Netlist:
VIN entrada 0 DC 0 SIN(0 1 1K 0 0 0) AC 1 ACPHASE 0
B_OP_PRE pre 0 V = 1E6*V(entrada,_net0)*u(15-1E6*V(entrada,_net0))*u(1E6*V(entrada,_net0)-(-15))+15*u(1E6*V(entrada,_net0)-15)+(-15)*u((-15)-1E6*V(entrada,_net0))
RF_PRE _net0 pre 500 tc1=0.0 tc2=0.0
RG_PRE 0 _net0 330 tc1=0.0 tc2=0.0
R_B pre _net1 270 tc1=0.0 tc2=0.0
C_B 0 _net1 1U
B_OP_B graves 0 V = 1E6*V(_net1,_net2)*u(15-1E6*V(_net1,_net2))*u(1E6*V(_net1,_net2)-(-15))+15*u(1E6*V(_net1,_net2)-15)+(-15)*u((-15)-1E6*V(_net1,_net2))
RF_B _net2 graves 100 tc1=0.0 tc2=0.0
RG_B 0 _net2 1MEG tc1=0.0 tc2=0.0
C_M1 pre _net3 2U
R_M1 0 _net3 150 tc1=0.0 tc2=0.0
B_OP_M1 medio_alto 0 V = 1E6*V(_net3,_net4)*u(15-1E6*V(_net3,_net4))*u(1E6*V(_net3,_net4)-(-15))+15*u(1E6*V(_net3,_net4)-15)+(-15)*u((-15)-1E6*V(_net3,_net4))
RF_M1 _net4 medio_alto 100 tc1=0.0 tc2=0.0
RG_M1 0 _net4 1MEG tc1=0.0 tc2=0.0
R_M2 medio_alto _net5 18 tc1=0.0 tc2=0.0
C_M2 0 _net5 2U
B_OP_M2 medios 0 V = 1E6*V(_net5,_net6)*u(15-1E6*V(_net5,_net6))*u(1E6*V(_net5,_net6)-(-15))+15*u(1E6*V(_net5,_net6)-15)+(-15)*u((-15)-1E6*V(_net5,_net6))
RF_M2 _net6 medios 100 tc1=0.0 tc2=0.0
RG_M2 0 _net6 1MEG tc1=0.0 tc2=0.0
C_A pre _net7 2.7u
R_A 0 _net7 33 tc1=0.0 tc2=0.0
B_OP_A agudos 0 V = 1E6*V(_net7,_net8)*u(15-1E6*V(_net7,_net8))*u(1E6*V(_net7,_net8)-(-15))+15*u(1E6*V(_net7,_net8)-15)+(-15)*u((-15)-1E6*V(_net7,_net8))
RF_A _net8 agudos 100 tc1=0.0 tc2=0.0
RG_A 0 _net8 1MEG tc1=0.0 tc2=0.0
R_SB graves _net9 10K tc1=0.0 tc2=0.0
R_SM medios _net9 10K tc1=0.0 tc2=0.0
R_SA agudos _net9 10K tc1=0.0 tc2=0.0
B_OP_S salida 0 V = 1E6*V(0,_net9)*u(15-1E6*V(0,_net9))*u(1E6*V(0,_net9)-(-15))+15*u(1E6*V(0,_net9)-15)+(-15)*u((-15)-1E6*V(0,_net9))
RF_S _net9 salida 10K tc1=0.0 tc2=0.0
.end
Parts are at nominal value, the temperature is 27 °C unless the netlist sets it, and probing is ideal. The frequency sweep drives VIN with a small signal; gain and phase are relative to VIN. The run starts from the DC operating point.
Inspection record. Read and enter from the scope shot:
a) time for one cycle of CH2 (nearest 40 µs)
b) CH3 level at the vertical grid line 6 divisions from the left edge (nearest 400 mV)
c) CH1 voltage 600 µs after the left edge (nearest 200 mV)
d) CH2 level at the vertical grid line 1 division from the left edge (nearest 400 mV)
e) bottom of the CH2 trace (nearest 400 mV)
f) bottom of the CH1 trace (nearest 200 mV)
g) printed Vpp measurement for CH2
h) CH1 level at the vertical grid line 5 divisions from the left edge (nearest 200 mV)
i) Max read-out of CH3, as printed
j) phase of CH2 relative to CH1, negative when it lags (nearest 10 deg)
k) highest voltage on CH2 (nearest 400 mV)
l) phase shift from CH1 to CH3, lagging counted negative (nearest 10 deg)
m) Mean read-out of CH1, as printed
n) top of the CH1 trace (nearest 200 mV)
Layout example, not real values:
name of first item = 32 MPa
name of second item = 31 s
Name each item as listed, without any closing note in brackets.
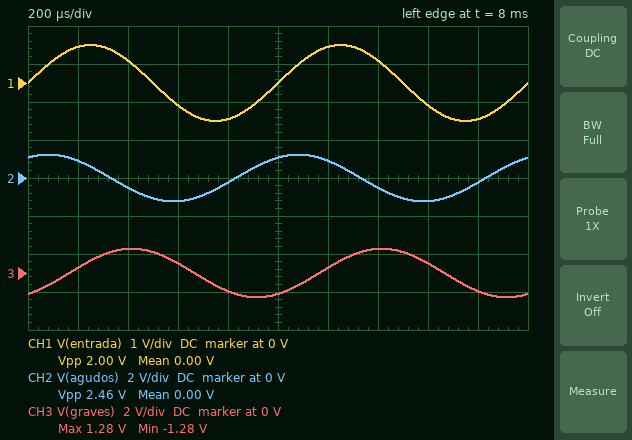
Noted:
time for one cycle of CH2 = 1.00 ms
CH3 level at the vertical grid line 6 divisions from the left edge = 400 mV
CH1 voltage 600 µs after the left edge = -600 mV
CH2 level at the vertical grid line 1 division from the left edge = 800 mV
bottom of the CH2 trace = -1.2 V
bottom of the CH1 trace = -1.0 V
printed Vpp measurement for CH2 = 2.46 V
CH1 level at the vertical grid line 5 divisions from the left edge = 0 V
Max read-out of CH3, as printed = 1.28 V
phase of CH2 relative to CH1, negative when it lags = 60 deg
highest voltage on CH2 = 1.2 V
phase shift from CH1 to CH3, lagging counted negative = -60 deg
Mean read-out of CH1, as printed = 0.00 V
top of the CH1 trace = 1.0 V
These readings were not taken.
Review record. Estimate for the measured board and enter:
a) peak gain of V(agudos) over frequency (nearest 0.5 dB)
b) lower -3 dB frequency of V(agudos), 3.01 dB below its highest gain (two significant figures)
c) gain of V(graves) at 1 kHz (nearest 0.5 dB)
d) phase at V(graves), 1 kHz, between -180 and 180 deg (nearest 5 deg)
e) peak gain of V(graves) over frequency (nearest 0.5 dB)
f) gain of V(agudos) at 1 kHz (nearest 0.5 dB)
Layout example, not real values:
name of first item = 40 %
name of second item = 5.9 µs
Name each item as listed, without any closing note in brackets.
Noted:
peak gain of V(agudos) over frequency = 8.0 dB
lower -3 dB frequency of V(agudos), 3.01 dB below its highest gain = 1.8 kHz
gain of V(graves) at 1 kHz = 2.0 dB
phase at V(graves), 1 kHz, between -180 and 180 deg = -60 deg
peak gain of V(graves) over frequency = 8.0 dB
gain of V(agudos) at 1 kHz = 2.0 dB
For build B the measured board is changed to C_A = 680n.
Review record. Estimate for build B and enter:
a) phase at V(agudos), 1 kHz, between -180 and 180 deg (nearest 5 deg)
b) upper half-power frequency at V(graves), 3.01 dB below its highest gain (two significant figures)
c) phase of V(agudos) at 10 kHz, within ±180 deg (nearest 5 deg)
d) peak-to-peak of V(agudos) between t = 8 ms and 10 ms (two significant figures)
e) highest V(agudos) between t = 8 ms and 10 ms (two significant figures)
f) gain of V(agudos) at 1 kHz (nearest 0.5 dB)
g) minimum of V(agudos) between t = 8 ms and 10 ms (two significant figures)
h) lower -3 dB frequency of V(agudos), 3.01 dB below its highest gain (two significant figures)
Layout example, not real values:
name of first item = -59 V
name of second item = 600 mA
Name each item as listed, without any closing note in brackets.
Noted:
phase at V(agudos), 1 kHz, between -180 and 180 deg = 80 deg
upper half-power frequency at V(graves), 3.01 dB below its highest gain = 590 Hz
phase of V(agudos) at 10 kHz, within ±180 deg = 35 deg
peak-to-peak of V(agudos) between t = 8 ms and 10 ms = 700 mV
highest V(agudos) between t = 8 ms and 10 ms = 350 mV
gain of V(agudos) at 1 kHz = -9.0 dB
minimum of V(agudos) between t = 8 ms and 10 ms = -350 mV
lower -3 dB frequency of V(agudos), 3.01 dB below its highest gain = 7.1 kHz
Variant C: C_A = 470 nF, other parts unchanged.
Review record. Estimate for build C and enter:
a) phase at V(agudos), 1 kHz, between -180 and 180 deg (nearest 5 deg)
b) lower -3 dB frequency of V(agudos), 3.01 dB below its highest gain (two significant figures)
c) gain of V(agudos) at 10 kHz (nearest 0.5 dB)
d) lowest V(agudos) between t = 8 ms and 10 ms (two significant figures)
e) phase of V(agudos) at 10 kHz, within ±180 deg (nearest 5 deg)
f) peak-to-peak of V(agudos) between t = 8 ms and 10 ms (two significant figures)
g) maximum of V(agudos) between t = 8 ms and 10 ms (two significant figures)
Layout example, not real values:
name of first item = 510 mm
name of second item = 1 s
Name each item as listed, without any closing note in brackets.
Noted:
phase at V(agudos), 1 kHz, between -180 and 180 deg = 85 deg
lower -3 dB frequency of V(agudos), 3.01 dB below its highest gain = 10 kHz
gain of V(agudos) at 10 kHz = 5.0 dB
lowest V(agudos) between t = 8 ms and 10 ms = -240 mV
phase of V(agudos) at 10 kHz, within ±180 deg = 45 deg
peak-to-peak of V(agudos) between t = 8 ms and 10 ms = 490 mV
maximum of V(agudos) between t = 8 ms and 10 ms = 240 mV
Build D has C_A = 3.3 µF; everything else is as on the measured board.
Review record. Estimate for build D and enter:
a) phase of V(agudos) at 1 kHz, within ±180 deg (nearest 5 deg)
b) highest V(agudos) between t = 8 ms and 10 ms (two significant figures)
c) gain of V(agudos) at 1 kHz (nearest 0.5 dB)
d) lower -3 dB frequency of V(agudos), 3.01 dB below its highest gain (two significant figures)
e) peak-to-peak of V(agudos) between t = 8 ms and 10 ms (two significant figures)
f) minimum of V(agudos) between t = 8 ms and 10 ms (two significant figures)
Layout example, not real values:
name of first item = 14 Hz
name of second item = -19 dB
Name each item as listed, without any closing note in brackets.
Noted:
phase of V(agudos) at 1 kHz, within ±180 deg = 55 deg
highest V(agudos) between t = 8 ms and 10 ms = 1.4 V
gain of V(agudos) at 1 kHz = 3.0 dB
lower -3 dB frequency of V(agudos), 3.01 dB below its highest gain = 1.5 kHz
peak-to-peak of V(agudos) between t = 8 ms and 10 ms = 2.8 V
minimum of V(agudos) between t = 8 ms and 10 ms = -1.4 V
